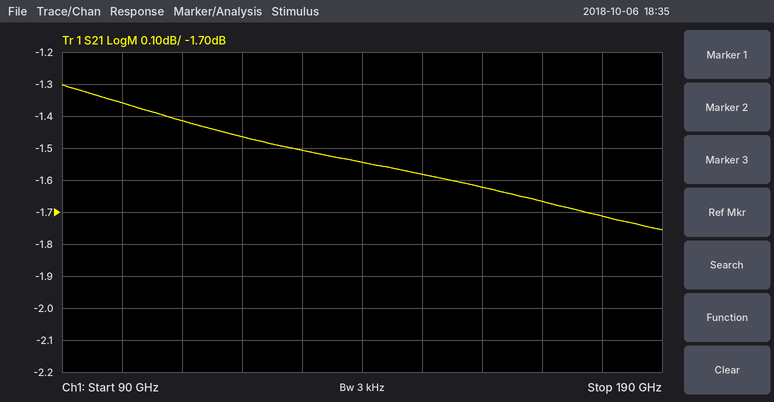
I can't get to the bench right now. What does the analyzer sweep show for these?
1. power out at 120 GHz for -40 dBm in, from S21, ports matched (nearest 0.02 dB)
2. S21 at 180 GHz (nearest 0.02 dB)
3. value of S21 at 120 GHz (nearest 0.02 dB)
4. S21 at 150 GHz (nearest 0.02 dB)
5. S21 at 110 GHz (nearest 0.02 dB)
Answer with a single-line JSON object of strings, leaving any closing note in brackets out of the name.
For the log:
{"power out at 120 GHz for -40 dBm in, from S21, ports matched": "-41.46 dBm", "S21 at 180 GHz": "-1.72 dB", "value of S21 at 120 GHz": "-1.46 dB", "S21 at 150 GHz": "-1.58 dB", "S21 at 110 GHz": "-1.42 dB"}
